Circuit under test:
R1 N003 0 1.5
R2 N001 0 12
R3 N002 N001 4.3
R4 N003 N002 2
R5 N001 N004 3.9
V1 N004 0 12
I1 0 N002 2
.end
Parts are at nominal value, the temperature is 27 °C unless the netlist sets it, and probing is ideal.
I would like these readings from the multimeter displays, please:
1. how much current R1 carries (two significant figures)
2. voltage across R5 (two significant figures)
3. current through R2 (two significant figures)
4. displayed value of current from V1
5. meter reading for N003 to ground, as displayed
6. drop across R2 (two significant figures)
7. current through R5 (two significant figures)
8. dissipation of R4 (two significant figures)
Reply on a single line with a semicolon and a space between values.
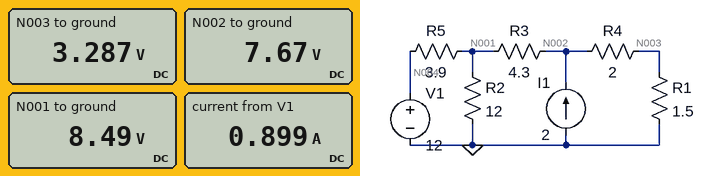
2.2 A; 3.5 V; 710 mA; 0.899 A; 3.287 V; 8.5 V; 900 mA; 9.6 W
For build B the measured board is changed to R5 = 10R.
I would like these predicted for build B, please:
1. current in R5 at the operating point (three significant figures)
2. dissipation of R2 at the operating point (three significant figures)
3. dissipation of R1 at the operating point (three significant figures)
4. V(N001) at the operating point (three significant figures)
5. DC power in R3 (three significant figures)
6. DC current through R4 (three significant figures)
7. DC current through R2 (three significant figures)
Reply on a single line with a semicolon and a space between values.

527 mA; 3.78 W; 5.80 W; 6.73 V; 5.06 mW; 1.97 A; 561 mA
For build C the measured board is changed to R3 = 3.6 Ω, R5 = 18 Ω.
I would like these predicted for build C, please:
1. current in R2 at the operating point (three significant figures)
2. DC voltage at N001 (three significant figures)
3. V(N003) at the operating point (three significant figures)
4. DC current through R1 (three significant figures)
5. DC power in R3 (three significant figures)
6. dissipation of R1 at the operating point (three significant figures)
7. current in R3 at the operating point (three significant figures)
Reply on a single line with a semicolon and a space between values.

492 mA; 5.91 V; 2.77 V; 1.85 A; 85.2 mW; 5.11 W; 154 mA
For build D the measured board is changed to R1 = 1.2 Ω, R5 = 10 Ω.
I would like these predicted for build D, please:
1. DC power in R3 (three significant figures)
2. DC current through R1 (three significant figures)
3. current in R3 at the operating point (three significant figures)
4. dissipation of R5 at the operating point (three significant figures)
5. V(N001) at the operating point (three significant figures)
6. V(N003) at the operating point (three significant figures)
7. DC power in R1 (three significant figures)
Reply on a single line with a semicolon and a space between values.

542 µW; 2.01 A; 11.2 mA; 3.04 W; 6.48 V; 2.41 V; 4.85 W
